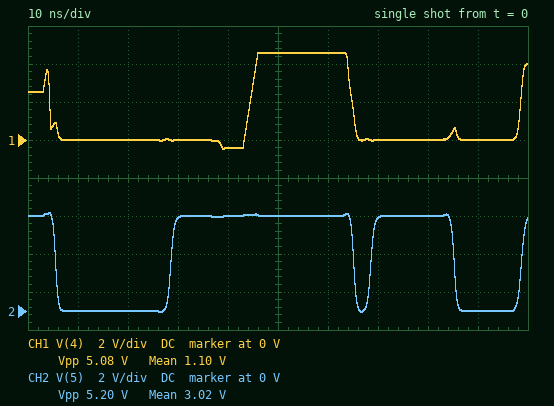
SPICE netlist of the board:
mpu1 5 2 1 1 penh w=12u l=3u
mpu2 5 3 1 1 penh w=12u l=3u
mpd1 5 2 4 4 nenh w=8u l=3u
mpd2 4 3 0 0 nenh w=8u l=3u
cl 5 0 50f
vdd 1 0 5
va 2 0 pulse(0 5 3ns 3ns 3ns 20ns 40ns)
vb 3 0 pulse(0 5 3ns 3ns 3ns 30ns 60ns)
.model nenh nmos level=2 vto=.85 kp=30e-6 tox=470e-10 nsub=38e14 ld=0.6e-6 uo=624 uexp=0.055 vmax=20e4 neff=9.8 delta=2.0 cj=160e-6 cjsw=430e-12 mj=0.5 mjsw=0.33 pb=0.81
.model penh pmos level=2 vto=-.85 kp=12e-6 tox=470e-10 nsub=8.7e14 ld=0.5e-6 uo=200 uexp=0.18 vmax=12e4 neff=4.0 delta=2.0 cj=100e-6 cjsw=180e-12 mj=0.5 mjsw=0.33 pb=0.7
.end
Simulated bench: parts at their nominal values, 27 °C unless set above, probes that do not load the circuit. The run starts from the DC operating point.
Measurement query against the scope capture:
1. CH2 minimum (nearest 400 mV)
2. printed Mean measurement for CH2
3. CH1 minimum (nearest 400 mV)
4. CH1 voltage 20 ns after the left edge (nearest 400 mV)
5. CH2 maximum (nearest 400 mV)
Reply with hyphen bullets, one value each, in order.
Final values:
- 0 V
- 3.02 V
- -400 mV
- 0 V
- 5.2 V
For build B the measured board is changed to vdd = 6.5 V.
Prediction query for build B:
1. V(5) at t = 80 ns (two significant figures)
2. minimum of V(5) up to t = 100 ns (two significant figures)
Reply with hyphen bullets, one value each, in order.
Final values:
- 6.5 V
- 110 mV
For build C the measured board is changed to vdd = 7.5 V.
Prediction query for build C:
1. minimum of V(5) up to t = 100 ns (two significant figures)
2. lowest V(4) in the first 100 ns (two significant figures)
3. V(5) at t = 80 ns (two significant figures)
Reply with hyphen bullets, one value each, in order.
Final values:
- 700 mV
- -470 mV
- 7.5 V
